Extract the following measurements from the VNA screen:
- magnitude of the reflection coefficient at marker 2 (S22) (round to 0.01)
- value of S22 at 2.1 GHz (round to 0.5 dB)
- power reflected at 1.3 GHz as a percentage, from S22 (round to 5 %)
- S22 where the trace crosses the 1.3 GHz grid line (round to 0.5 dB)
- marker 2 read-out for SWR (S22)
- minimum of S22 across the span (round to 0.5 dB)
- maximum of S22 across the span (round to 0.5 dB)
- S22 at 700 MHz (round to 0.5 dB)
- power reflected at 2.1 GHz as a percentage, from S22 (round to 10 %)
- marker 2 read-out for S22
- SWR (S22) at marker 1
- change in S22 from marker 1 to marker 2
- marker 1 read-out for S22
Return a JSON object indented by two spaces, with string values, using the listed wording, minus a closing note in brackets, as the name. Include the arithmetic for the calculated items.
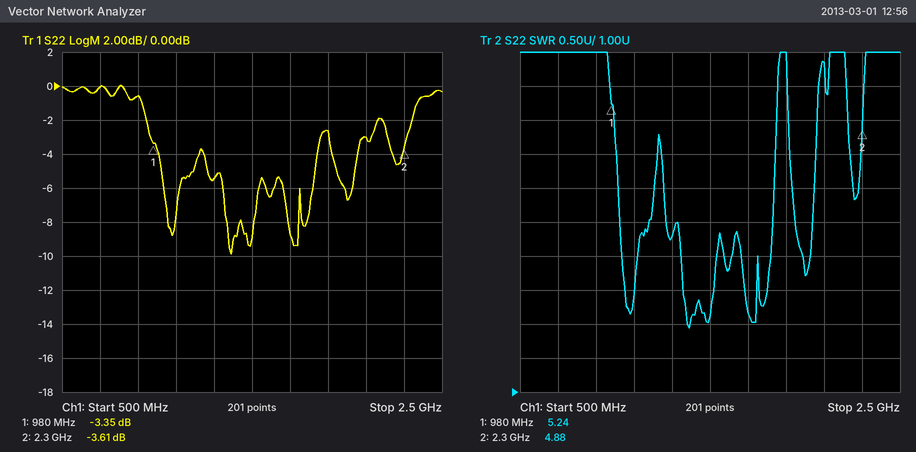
{
  "magnitude of the reflection coefficient at marker 2 (S22)": "10^(-3.61/20) ≈ 0.66",
  "value of S22 at 2.1 GHz": "-3.0 dB",
  "power reflected at 1.3 GHz as a percentage, from S22": "10^(-5.5/10) ≈ 28.2 %, so 30 % to the nearest 5 %",
  "S22 where the trace crosses the 1.3 GHz grid line": "-5.5 dB",
  "marker 2 read-out for SWR": "4.88",
  "minimum of S22 across the span": "-10.0 dB",
  "maximum of S22 across the span": "0.0 dB",
  "S22 at 700 MHz": "0.0 dB",
  "power reflected at 2.1 GHz as a percentage, from S22": "10^(-3/10) ≈ 50 %",
  "marker 2 read-out for S22": "-3.61 dB",
  "SWR (S22) at marker 1": "5.24",
  "change in S22 from marker 1 to marker 2": "-3.61 − (-3.35) = -0.26 dB",
  "marker 1 read-out for S22": "-3.35 dB"
}
